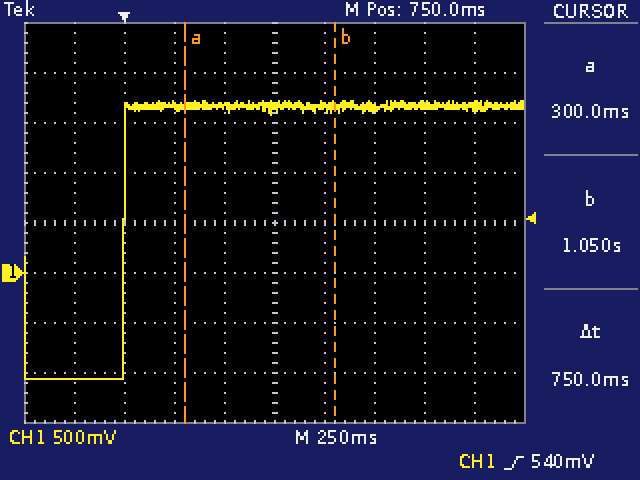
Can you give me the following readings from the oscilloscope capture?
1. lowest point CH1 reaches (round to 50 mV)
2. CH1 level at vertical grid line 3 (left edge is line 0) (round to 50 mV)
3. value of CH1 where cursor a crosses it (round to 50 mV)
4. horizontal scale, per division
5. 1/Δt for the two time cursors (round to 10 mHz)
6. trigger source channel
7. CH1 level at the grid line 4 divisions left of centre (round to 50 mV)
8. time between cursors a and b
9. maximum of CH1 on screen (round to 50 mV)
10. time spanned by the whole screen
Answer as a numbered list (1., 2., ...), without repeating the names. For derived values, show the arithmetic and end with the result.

1. -1.05 V
2. 1.65 V
3. 1.65 V
4. 250 ms
5. 1 / 750 ms ≈ 1.33 Hz
6. CH1
7. -1.05 V
8. 750 ms
9. 1.70 V
10. 2.5 s
